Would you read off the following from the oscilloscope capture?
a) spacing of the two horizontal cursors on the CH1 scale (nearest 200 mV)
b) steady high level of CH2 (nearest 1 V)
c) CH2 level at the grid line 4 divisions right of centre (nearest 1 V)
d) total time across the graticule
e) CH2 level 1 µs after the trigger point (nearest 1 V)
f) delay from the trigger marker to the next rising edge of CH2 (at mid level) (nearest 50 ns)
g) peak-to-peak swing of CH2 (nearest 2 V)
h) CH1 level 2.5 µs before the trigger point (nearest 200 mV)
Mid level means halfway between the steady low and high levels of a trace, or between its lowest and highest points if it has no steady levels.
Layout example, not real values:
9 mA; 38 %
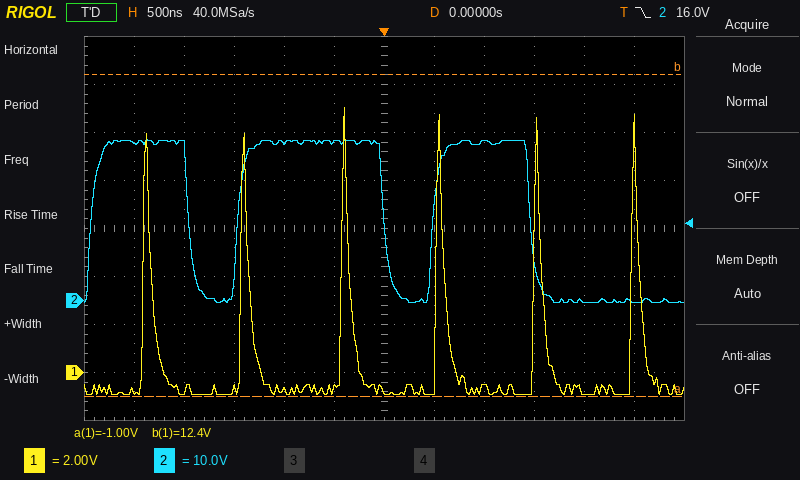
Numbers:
13.4 V; 33 V; 0 V; 6 µs; 33 V; 500 ns; 34 V; -800 mV
